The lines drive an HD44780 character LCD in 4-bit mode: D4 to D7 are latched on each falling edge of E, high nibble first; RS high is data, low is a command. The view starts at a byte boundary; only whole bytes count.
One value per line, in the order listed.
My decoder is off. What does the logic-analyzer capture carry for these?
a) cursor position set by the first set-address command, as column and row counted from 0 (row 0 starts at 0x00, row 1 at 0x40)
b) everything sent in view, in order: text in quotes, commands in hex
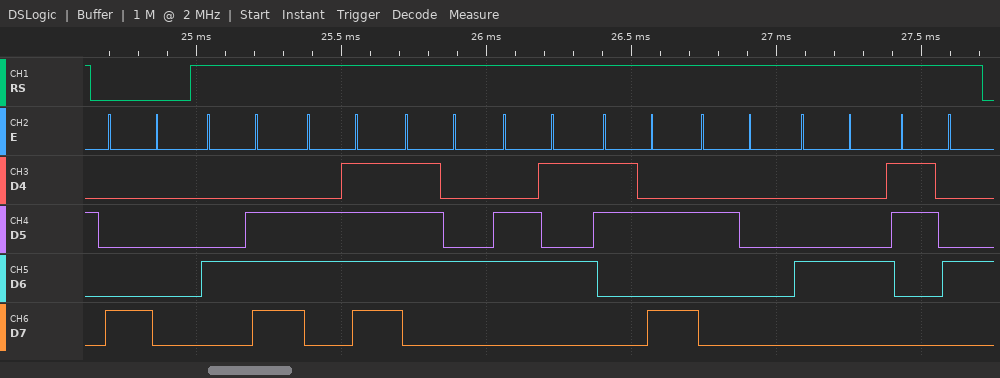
column 0, row 0
0x80 "Note: D4"
